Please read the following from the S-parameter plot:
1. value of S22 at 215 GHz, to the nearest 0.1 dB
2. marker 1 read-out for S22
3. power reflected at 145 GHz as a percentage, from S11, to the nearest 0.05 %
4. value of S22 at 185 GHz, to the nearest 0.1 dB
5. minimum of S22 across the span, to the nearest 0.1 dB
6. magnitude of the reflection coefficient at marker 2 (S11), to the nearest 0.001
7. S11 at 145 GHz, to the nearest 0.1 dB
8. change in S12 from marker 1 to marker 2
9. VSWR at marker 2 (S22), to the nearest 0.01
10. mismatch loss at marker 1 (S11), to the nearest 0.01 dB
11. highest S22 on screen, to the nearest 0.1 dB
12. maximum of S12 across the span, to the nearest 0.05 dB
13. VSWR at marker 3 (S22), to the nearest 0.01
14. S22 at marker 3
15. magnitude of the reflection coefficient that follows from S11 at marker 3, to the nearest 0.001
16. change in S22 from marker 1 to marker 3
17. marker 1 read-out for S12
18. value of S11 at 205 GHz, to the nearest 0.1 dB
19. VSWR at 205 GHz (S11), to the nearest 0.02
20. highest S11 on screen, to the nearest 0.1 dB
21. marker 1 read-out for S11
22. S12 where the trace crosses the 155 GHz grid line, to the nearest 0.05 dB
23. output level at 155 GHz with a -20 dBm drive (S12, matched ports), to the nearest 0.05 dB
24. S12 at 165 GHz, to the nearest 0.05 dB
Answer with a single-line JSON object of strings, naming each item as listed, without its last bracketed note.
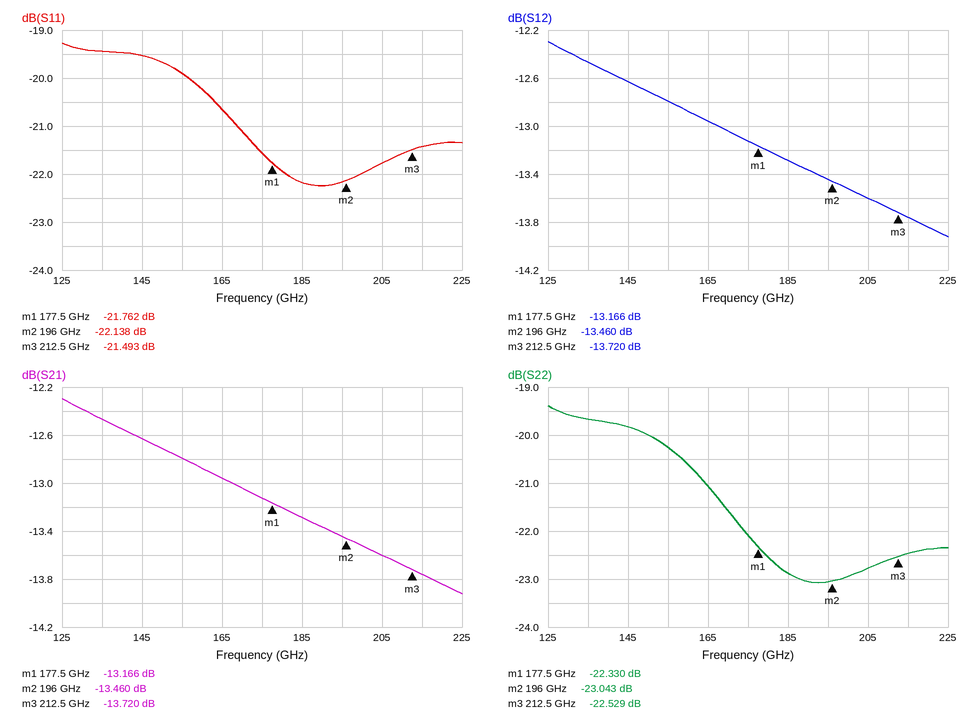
{"value of S22 at 215 GHz, to the nearest 0.1 dB": "-22.5 dB", "marker 1 read-out for S22": "-22.330 dB", "power reflected at 145 GHz as a percentage, from S11, to the nearest 0.05 %": "1.10 %", "value of S22 at 185 GHz, to the nearest 0.1 dB": "-22.9 dB", "minimum of S22 across the span, to the nearest 0.1 dB": "-23.1 dB", "magnitude of the reflection coefficient at marker 2 (S11), to the nearest 0.001": "0.078", "S11 at 145 GHz, to the nearest 0.1 dB": "-19.5 dB", "change in S12 from marker 1 to marker 2": "-0.294 dB", "VSWR at marker 2 (S22), to the nearest 0.01": "1.15", "mismatch loss at marker 1 (S11), to the nearest 0.01 dB": "0.03 dB", "highest S22 on screen, to the nearest 0.1 dB": "-19.4 dB", "maximum of S12 across the span, to the nearest 0.05 dB": "-12.30 dB", "VSWR at marker 3 (S22), to the nearest 0.01": "1.16", "S22 at marker 3": "-22.529 dB", "magnitude of the reflection coefficient that follows from S11 at marker 3, to the nearest 0.001": "0.084", "change in S22 from marker 1 to marker 3": "-0.199 dB", "marker 1 read-out for S12": "-13.166 dB", "value of S11 at 205 GHz, to the nearest 0.1 dB": "-21.8 dB", "VSWR at 205 GHz (S11), to the nearest 0.02": "1.18", "highest S11 on screen, to the nearest 0.1 dB": "-19.3 dB", "marker 1 read-out for S11": "-21.762 dB", "S12 where the trace crosses the 155 GHz grid line, to the nearest 0.05 dB": "-12.80 dB", "output level at 155 GHz with a -20 dBm drive (S12, matched ports), to the nearest 0.05 dB": "-32.80 dBm", "S12 at 165 GHz, to the nearest 0.05 dB": "-12.95 dB"}
